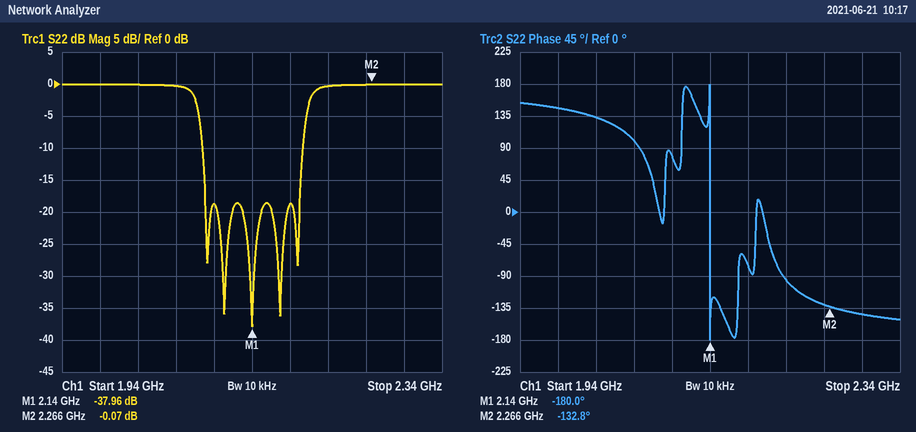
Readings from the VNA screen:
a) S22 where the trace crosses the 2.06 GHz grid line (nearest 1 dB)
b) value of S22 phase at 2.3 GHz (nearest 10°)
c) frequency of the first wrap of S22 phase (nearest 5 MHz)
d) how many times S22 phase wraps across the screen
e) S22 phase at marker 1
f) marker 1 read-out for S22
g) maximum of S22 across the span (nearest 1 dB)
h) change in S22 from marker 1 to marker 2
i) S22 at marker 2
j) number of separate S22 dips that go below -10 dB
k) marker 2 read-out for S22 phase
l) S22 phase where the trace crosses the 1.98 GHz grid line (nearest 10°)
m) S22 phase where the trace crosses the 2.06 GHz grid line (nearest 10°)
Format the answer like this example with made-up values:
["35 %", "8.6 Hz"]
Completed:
["0 dB", "-140°", "2.140 GHz", "1", "-180.0°", "-37.96 dB", "0 dB", "37.89 dB", "-0.07 dB", "5", "-132.8°", "150°", "100°"]
